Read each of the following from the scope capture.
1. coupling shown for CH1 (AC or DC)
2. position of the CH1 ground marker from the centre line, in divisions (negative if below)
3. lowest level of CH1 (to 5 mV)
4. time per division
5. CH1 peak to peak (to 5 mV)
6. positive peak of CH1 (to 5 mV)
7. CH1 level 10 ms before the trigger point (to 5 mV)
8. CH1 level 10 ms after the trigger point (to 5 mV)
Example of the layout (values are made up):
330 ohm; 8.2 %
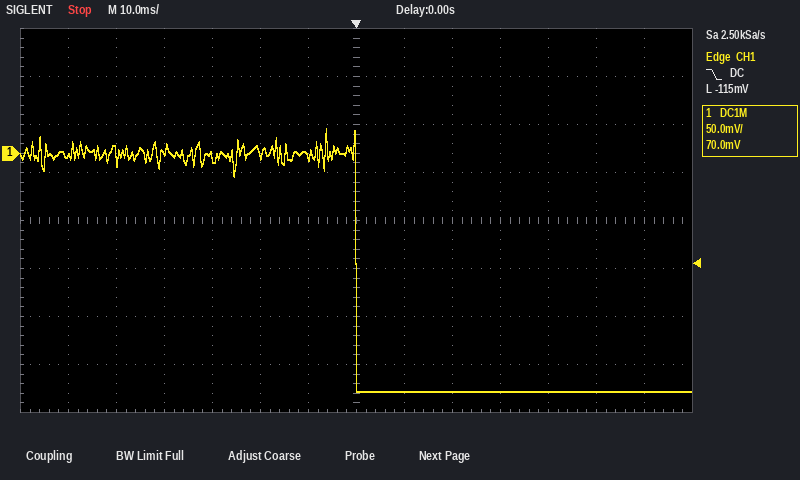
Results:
DC; +1.4 div; -250 mV; 10 ms; 275 mV; 25 mV; -5 mV; -250 mV
